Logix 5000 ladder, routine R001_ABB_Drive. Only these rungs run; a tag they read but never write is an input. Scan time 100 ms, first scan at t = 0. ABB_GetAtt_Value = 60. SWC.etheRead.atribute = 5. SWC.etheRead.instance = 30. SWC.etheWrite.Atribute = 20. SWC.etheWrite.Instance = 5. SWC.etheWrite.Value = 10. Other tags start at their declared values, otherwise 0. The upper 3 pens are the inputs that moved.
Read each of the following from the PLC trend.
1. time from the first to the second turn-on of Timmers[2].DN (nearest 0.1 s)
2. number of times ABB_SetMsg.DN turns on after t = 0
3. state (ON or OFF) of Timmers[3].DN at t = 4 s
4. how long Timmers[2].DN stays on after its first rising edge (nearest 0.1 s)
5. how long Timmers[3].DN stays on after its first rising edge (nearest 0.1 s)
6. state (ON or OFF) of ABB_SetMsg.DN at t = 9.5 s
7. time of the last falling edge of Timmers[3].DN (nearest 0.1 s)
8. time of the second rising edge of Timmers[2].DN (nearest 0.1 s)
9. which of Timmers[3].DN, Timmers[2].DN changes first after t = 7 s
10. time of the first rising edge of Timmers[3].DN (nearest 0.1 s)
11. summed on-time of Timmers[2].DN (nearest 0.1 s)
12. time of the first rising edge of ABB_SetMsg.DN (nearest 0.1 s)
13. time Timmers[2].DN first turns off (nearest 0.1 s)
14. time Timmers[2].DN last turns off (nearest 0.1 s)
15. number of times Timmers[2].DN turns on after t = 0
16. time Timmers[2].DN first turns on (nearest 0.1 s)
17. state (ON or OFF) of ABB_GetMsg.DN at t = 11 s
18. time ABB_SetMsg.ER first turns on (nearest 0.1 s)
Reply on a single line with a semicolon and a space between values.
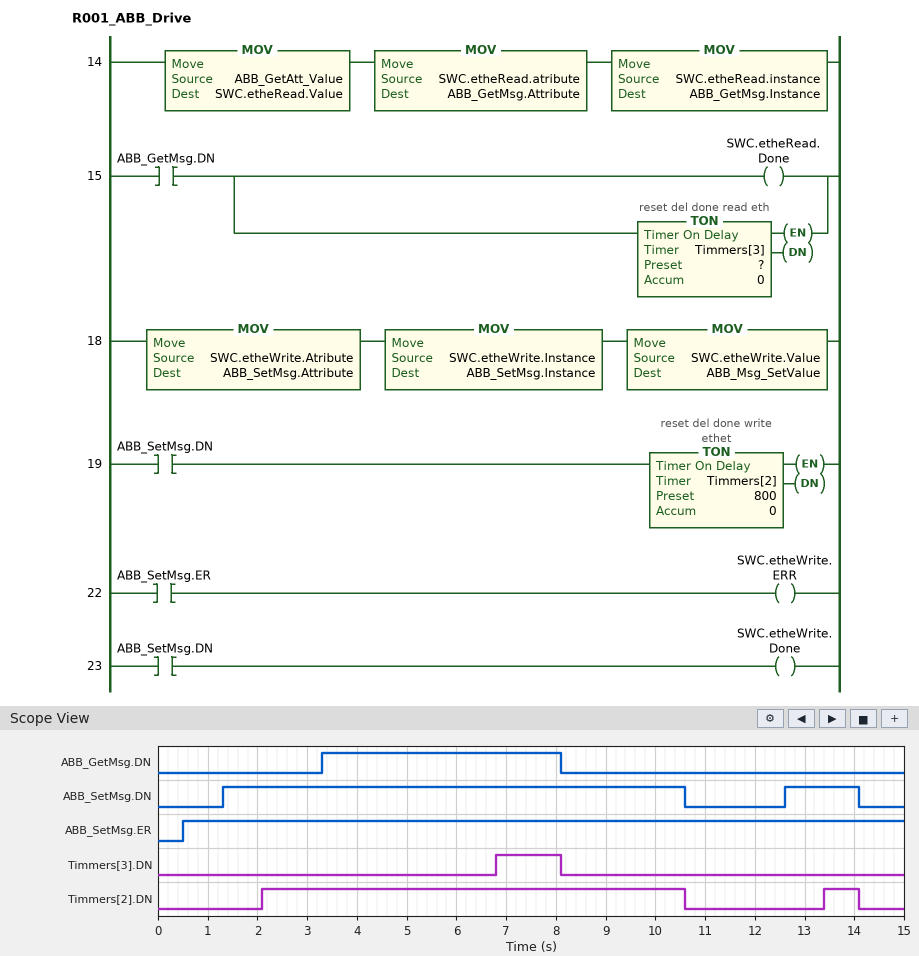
11.3 s; 2; OFF; 8.5 s; 1.3 s; ON; 8.1 s; 13.4 s; Timmers[3].DN; 6.8 s; 9.2 s; 1.3 s; 10.6 s; 14.1 s; 2; 2.1 s; OFF; 0.5 s
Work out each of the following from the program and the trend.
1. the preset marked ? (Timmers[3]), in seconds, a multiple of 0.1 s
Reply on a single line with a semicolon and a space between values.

3.5 s
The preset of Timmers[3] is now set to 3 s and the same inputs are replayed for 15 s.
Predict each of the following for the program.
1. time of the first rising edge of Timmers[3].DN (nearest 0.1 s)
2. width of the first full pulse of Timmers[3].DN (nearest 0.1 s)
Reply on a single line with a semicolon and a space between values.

6.3 s; 1.8 s
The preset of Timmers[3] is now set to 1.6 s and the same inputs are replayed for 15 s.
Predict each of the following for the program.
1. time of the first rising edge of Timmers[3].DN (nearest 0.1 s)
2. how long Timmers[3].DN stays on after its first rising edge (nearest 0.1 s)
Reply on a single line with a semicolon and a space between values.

4.9 s; 3.2 s
